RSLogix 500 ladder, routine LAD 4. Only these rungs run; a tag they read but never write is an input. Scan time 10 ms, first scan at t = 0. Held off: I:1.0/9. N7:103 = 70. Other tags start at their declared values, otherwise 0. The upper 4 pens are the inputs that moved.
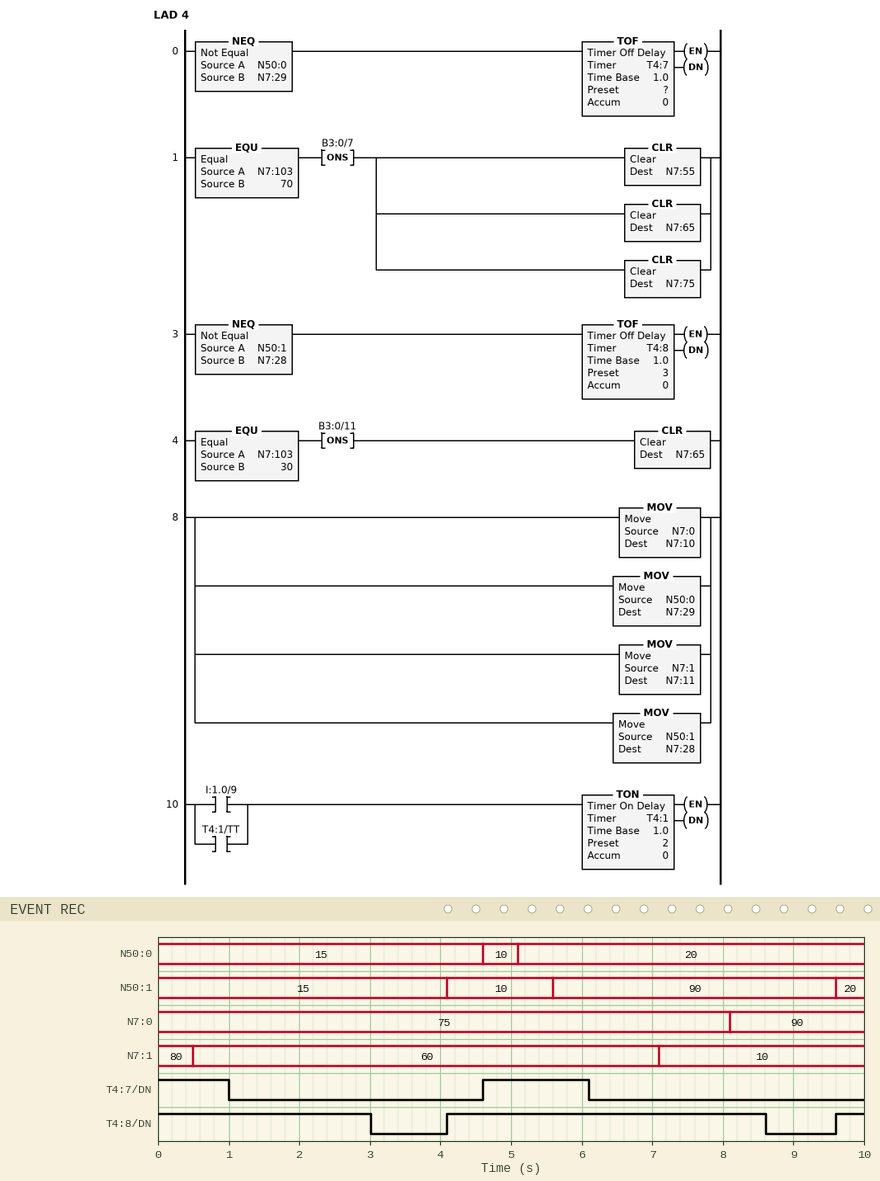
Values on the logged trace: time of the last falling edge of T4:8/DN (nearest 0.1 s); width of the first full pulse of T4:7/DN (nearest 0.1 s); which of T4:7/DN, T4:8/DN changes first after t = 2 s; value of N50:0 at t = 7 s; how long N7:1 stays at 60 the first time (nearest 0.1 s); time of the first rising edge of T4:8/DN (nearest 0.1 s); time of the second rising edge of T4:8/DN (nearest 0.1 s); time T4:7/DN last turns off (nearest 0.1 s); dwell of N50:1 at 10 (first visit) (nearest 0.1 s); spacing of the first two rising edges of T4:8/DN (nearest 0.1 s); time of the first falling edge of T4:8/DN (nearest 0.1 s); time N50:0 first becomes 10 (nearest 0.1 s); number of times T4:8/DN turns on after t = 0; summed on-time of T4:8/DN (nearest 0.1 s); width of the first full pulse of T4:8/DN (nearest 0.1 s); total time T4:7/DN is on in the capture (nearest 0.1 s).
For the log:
8.6 s
1.5 s
T4:8/DN
20
6.6 s
4.1 s
9.6 s
6.1 s
1.5 s
5.5 s
3.0 s
4.6 s
2
7.9 s
4.5 s
2.5 s
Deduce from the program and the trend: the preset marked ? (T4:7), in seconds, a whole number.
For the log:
1 s
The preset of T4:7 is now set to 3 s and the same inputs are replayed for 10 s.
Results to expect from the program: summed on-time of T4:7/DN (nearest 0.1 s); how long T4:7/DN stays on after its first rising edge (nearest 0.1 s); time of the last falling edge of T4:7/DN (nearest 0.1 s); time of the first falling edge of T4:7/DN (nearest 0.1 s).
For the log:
6.5 s
3.5 s
8.1 s
3.0 s
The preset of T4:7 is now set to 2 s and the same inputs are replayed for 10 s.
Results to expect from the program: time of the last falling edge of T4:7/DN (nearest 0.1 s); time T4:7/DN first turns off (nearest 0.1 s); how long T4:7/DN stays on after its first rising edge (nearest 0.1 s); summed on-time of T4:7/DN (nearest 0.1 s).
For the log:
7.1 s
2.0 s
2.5 s
4.5 s
